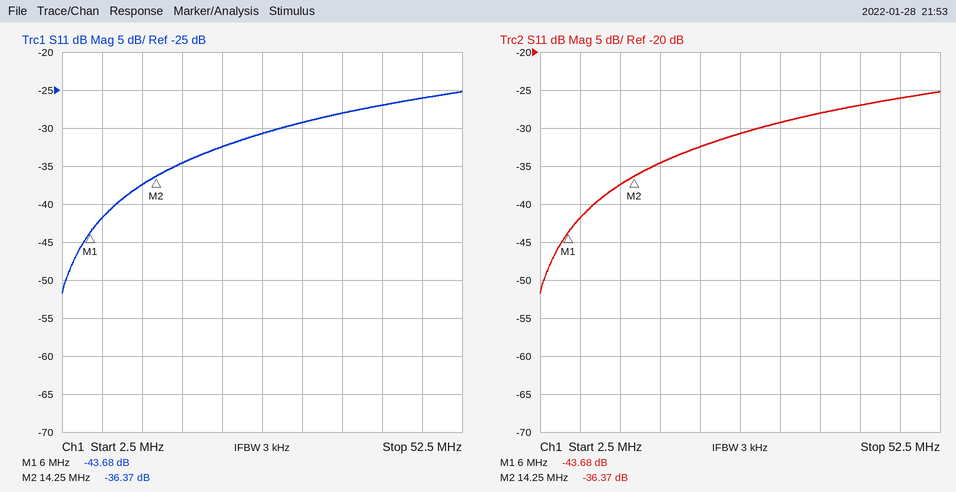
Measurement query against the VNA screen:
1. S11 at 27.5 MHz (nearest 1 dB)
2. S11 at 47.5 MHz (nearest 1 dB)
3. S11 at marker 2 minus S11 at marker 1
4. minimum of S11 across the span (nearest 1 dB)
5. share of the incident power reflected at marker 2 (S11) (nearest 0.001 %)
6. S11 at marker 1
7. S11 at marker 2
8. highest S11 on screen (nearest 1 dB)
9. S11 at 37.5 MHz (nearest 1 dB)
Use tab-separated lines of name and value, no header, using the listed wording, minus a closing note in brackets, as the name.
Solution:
S11 at 27.5 MHz	-31 dB
S11 at 47.5 MHz	-26 dB
S11 at marker 2 minus S11 at marker 1	7.31 dB
minimum of S11 across the span	-52 dB
share of the incident power reflected at marker 2 (S11)	0.023 %
S11 at marker 1	-43.68 dB
S11 at marker 2	-36.37 dB
highest S11 on screen	-25 dB
S11 at 37.5 MHz	-28 dB
